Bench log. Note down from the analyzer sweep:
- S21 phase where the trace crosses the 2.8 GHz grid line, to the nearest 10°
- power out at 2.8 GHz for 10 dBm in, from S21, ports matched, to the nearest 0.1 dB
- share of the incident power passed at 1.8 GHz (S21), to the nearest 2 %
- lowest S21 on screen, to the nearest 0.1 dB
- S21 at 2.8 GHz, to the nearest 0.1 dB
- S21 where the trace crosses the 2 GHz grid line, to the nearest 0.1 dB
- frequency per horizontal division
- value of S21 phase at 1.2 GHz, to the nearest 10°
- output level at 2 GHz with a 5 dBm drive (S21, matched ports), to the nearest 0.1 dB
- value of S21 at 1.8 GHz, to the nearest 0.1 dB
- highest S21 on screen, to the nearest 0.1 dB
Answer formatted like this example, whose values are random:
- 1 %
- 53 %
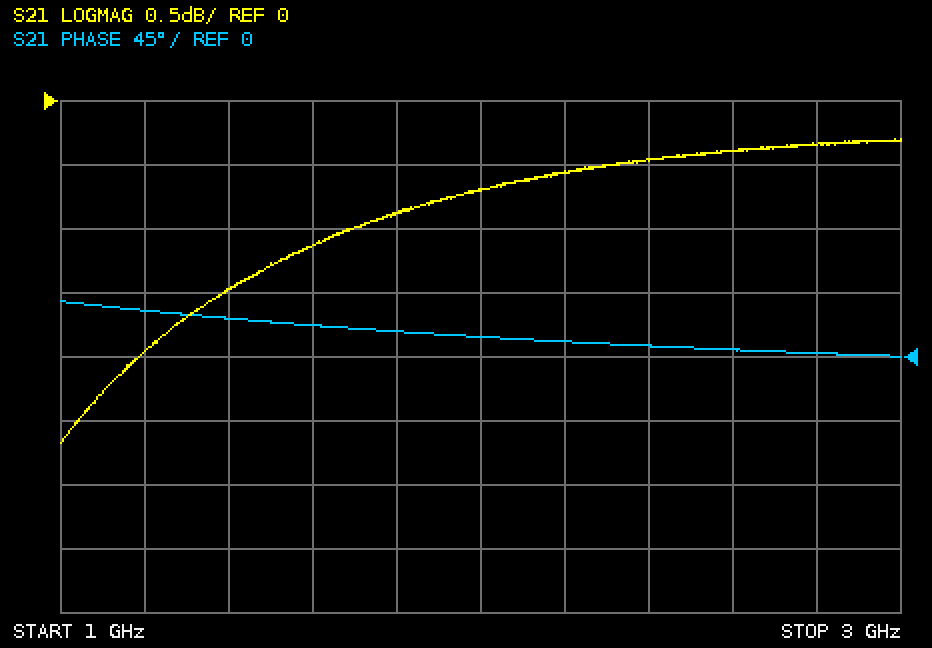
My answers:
- 0°
- 9.7 dBm
- 82 %
- -2.7 dB
- -0.3 dB
- -0.7 dB
- 200 MHz
- 30°
- 4.3 dBm
- -0.9 dB
- -0.3 dB
